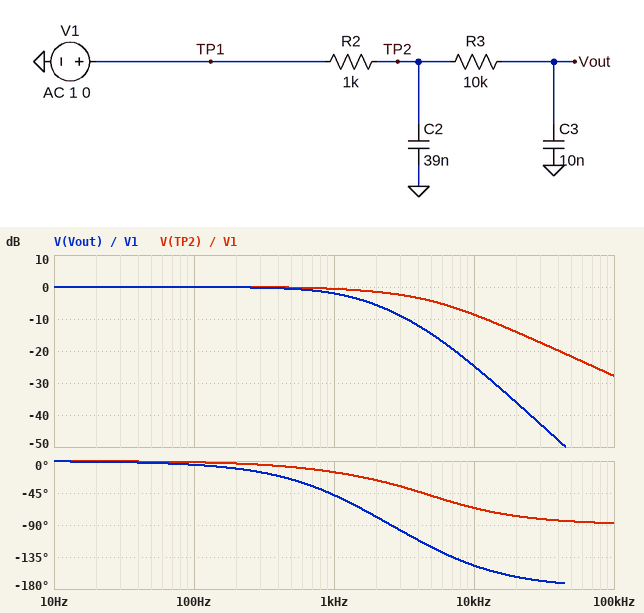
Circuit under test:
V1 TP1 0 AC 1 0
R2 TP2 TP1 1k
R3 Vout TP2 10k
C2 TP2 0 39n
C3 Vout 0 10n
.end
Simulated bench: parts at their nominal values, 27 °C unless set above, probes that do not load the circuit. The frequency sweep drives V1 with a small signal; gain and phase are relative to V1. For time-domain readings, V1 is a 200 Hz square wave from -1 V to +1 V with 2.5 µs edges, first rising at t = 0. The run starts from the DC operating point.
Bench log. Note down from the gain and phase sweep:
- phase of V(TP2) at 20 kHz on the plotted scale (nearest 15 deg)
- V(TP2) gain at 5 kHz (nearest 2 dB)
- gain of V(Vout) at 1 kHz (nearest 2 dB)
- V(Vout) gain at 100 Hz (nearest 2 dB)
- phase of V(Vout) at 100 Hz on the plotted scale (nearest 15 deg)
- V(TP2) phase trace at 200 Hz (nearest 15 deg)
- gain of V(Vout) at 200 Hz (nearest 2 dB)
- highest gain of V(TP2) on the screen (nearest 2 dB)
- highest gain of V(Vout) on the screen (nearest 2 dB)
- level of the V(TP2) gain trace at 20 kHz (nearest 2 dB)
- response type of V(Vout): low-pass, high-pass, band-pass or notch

-75 deg
-4 dB
-2 dB
0 dB
0 deg
0 deg
0 dB
0 dB
0 dB
-14 dB
low-pass
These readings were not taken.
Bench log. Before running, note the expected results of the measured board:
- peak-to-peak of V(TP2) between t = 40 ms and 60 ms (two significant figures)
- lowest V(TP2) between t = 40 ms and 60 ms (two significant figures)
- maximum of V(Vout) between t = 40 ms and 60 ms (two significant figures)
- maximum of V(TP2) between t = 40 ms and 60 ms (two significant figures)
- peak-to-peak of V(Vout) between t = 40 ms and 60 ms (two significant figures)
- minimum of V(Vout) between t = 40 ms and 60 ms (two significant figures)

2.0 V
-1.0 V
1.0 V
1.0 V
2.0 V
-1.0 V
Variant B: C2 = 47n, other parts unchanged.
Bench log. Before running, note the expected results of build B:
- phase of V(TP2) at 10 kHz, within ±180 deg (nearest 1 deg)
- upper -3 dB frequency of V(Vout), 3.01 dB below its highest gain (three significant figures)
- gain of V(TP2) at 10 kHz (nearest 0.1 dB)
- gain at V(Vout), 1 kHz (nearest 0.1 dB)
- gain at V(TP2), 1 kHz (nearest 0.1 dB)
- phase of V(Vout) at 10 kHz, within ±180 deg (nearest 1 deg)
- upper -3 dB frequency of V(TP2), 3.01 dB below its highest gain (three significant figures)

-70 deg
1.24 kHz
-10.0 dB
-2.1 dB
-0.7 dB
-151 deg
2.96 kHz
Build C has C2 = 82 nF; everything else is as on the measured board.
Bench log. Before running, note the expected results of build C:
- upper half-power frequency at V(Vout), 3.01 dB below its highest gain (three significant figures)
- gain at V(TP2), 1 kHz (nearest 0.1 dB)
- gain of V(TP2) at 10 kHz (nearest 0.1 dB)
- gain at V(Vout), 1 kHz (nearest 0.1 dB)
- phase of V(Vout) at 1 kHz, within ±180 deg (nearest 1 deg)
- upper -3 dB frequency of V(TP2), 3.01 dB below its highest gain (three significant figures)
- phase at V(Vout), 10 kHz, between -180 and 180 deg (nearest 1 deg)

1.04 kHz
-1.4 dB
-14.5 dB
-2.8 dB
-61 deg
1.73 kHz
-159 deg
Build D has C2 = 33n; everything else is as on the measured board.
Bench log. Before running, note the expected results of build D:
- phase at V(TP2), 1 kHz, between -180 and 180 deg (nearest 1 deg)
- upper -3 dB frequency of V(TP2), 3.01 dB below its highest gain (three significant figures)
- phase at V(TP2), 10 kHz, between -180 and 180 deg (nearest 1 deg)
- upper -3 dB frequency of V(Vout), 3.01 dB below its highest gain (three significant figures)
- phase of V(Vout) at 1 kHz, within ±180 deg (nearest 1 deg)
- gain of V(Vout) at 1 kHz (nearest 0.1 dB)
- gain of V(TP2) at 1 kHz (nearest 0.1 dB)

-14 deg
4.20 kHz
-62 deg
1.32 kHz
-46 deg
-1.9 dB
-0.5 dB
